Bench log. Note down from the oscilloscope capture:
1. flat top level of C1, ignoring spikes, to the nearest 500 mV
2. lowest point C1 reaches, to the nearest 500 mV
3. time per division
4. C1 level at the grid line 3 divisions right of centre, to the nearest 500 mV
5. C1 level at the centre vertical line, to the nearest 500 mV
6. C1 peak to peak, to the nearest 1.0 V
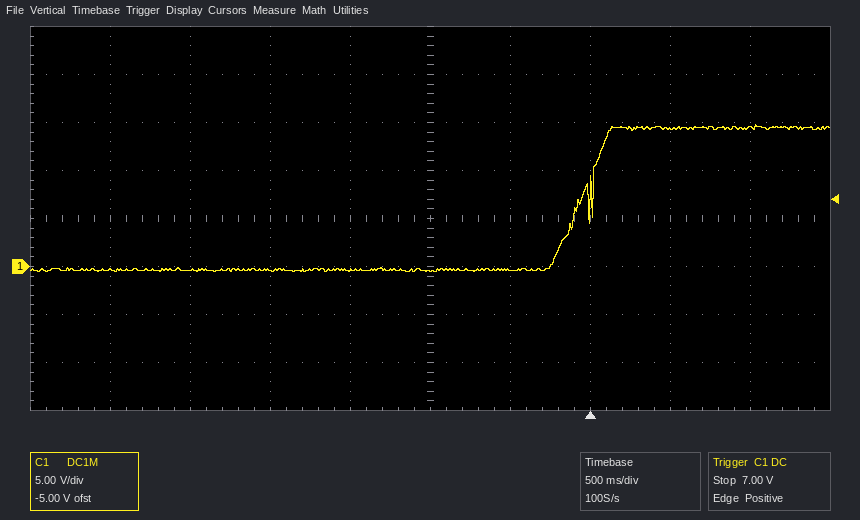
14.5 V
-500 mV
500 ms
14.5 V
-500 mV
15.0 V
